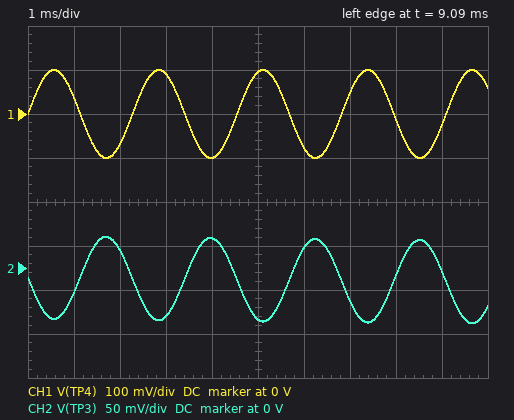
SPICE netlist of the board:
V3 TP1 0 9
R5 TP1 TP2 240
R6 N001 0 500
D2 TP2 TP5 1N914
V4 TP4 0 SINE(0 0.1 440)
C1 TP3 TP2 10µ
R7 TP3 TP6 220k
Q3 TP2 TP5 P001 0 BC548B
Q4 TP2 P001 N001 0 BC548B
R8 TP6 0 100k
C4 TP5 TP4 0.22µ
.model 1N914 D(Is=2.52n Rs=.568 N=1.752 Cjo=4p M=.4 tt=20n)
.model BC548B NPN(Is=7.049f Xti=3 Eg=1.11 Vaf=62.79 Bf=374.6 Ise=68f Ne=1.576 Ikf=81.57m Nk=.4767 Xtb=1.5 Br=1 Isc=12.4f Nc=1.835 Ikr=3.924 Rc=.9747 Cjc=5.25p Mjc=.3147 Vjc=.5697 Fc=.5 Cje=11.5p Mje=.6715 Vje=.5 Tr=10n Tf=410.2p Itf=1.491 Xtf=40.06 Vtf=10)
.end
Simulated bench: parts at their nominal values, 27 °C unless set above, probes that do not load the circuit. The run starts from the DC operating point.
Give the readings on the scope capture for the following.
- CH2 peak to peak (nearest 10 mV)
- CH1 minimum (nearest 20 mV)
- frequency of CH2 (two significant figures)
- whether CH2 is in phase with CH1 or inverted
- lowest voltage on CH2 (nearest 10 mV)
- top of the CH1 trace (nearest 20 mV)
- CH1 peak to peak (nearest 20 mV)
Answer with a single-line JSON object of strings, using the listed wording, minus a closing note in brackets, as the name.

{"CH2 peak to peak": "100 mV", "CH1 minimum": "-100 mV", "frequency of CH2": "440 Hz", "whether CH2 is in phase with CH1 or inverted": "inverted", "lowest voltage on CH2": "-60 mV", "top of the CH1 trace": "100 mV", "CH1 peak to peak": "200 mV"}
